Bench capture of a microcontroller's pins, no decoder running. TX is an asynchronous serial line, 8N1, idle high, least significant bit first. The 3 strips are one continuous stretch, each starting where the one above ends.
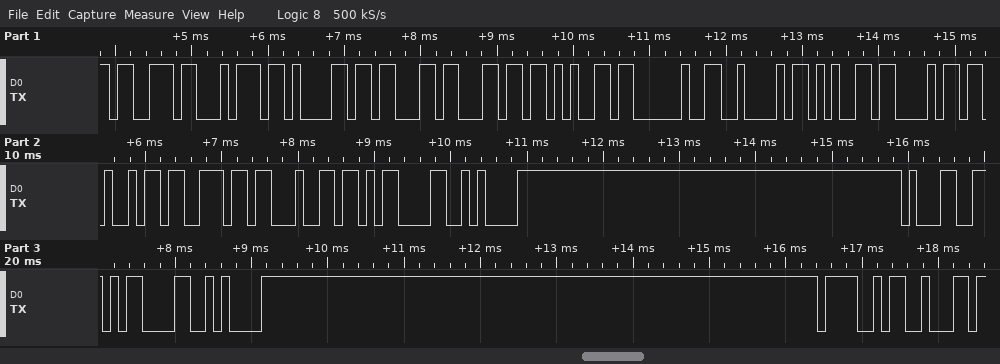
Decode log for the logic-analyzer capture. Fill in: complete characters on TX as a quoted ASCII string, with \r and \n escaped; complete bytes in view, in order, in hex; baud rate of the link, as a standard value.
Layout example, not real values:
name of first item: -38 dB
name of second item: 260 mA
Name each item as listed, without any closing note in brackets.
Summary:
complete characters on TX as a quoted ASCII string, with \r and \n escaped: "stacle Behind\r\n1\r\nOb"
complete bytes in view, in order, in hex: 73 74 61 63 6C 65 20 42 65 68 69 6E 64 0D 0A 31 0D 0A 4F 62
baud rate of the link, as a standard value: 9600 baud
